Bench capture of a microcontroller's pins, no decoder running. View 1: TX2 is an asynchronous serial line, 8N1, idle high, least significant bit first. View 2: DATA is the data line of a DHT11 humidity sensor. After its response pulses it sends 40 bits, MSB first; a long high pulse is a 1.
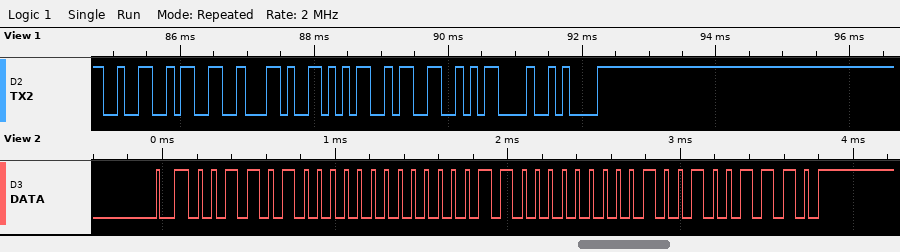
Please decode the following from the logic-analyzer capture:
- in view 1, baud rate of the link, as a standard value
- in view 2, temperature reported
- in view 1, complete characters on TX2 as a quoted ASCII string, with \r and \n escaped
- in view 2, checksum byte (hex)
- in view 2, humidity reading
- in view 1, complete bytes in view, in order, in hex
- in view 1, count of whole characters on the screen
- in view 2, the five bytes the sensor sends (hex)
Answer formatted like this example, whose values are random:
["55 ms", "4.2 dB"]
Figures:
["9600 baud", "24.2 °C", "\"23,53\\r\\n\"", "0x4E", "52 %", "32 33 2C 35 33 0D 0A", "7", "34 00 18 02 4E"]
